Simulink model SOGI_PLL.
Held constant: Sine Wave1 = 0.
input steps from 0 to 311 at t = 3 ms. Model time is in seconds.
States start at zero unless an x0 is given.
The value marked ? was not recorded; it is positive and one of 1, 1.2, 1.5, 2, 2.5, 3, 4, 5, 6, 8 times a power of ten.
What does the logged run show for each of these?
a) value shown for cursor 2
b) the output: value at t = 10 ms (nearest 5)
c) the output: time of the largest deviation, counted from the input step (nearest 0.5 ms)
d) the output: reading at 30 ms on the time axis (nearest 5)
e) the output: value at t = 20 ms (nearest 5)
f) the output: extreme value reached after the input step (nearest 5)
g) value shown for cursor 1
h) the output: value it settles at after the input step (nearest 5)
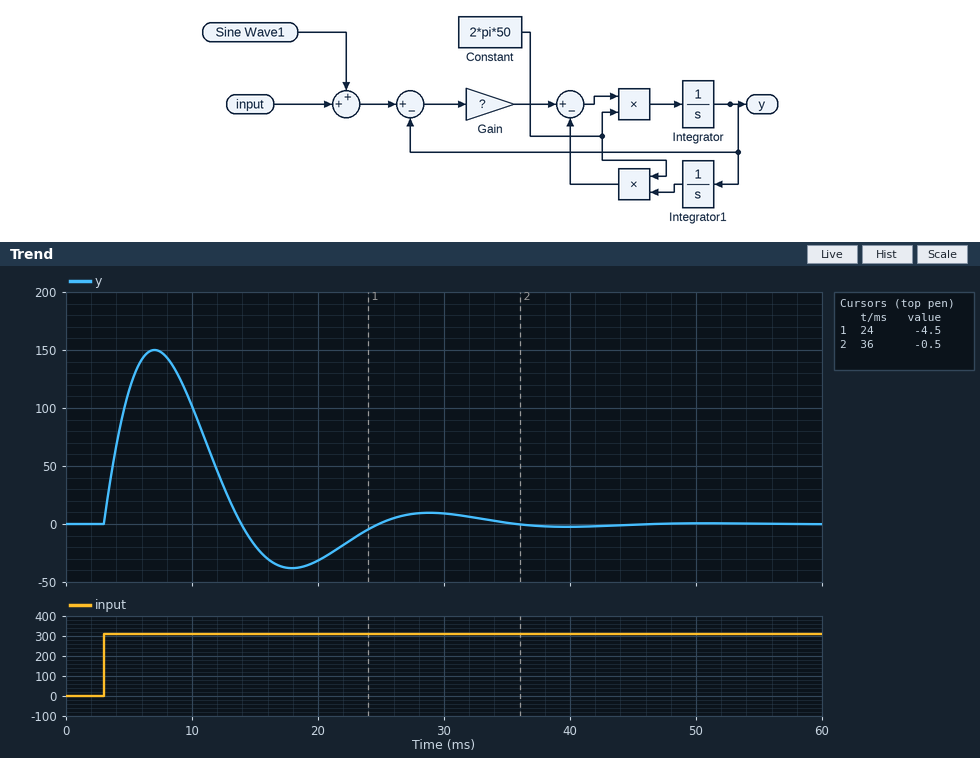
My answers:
-0.5
100
4.0 ms
10
-30
150
-4.5
0
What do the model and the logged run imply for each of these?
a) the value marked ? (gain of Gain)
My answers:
0.8
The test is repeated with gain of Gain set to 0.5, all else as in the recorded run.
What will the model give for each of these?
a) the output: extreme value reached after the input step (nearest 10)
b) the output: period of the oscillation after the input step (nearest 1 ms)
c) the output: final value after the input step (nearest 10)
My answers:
110
21 ms
0
